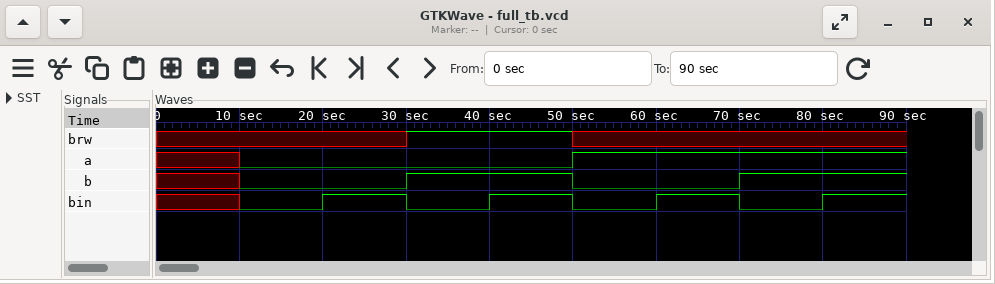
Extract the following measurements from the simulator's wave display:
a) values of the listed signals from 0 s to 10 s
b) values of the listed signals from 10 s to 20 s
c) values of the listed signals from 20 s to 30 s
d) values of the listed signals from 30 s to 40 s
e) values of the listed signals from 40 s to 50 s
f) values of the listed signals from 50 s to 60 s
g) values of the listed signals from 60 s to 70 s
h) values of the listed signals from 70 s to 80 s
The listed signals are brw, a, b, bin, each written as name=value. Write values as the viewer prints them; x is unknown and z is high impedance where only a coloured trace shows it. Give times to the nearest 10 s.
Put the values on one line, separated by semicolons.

brw=x, a=x, b=x, bin=x; brw=x, a=0, b=0, bin=0; brw=x, a=0, b=0, bin=1; brw=1, a=0, b=1, bin=0; brw=1, a=0, b=1, bin=1; brw=x, a=1, b=0, bin=0; brw=x, a=1, b=0, bin=1; brw=x, a=1, b=1, bin=0
